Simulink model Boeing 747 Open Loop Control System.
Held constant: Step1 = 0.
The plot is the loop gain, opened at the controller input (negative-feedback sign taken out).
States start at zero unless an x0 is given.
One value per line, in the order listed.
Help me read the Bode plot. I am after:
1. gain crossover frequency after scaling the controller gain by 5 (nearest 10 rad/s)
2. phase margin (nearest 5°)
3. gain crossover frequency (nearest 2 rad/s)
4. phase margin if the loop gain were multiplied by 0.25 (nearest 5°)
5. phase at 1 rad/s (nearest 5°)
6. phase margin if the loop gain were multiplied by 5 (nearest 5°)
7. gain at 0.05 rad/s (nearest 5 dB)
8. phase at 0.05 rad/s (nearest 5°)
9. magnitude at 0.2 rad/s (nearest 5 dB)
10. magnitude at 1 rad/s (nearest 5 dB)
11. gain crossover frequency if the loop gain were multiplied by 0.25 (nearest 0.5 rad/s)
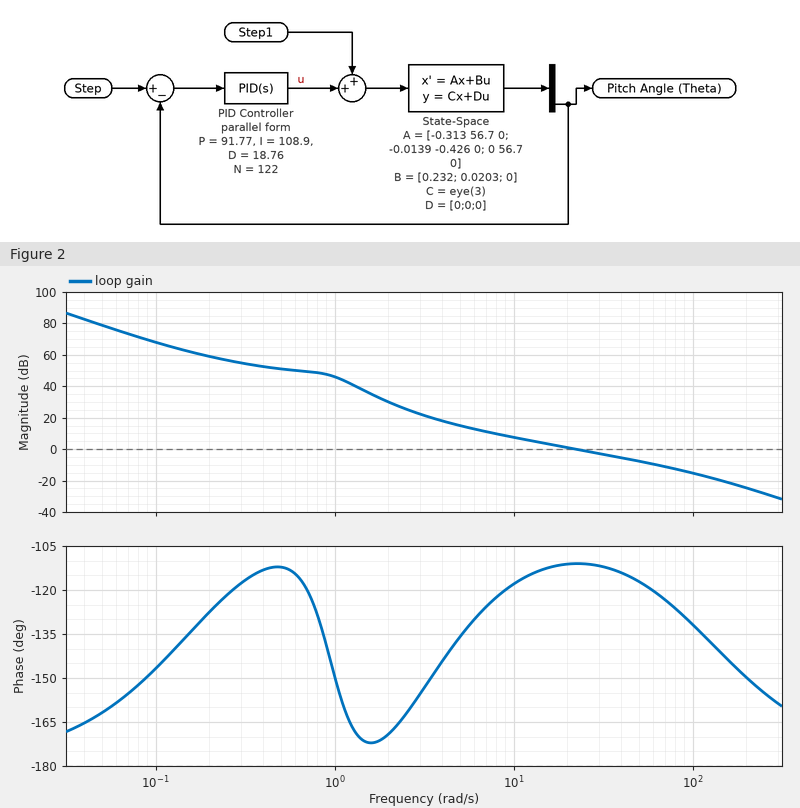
90 rad/s
70°
22 rad/s
50°
-150°
50°
80 dB
-160°
60 dB
45 dB
6.5 rad/s
